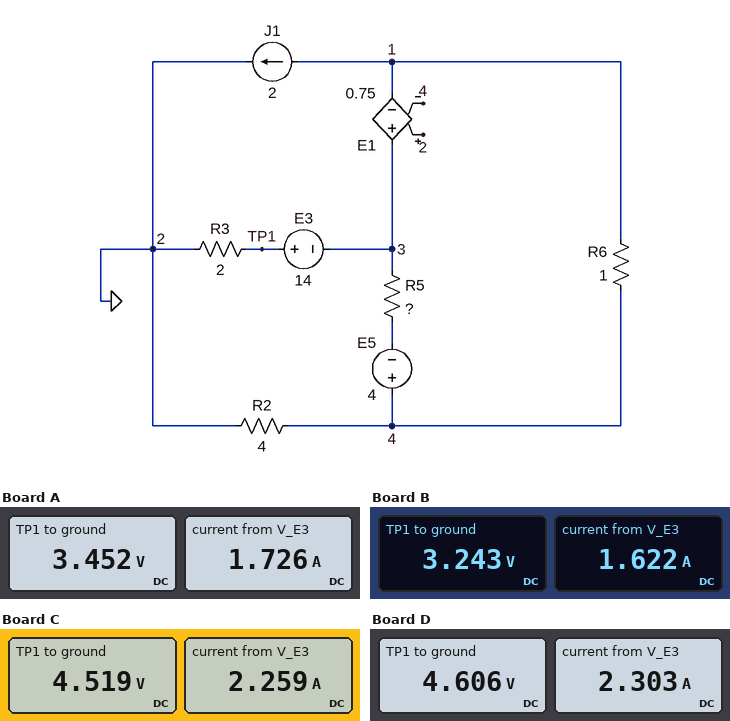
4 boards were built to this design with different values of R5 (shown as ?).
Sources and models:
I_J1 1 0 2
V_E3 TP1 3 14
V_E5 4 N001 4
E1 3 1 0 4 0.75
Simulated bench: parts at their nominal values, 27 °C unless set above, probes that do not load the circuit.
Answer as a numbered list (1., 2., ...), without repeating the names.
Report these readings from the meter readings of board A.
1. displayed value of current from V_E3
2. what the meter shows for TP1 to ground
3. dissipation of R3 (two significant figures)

1. 1.726 A
2. 3.452 V
3. 6.0 W
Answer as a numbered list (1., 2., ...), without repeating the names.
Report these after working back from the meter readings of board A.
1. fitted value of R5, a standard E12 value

1. 2.7 Ω
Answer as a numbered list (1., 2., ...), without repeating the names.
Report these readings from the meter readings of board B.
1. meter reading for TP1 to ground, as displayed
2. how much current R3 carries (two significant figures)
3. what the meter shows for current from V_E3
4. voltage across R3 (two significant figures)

1. 3.243 V
2. 1.6 A
3. 1.622 A
4. 3.2 V
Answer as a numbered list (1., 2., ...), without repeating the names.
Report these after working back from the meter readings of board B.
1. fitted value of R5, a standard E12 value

1. 2.2 Ω
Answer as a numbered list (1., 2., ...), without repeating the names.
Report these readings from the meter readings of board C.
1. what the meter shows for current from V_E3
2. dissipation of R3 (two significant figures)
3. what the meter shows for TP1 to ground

1. 2.259 A
2. 10 W
3. 4.519 V
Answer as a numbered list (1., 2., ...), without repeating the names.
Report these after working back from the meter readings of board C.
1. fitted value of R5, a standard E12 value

1. 12 Ω
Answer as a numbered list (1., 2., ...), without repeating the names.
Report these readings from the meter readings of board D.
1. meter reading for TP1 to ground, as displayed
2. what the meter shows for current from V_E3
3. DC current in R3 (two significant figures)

1. 4.606 V
2. 2.303 A
3. 2.3 A
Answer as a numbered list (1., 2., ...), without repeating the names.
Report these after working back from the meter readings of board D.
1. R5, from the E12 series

1. 15 Ω
